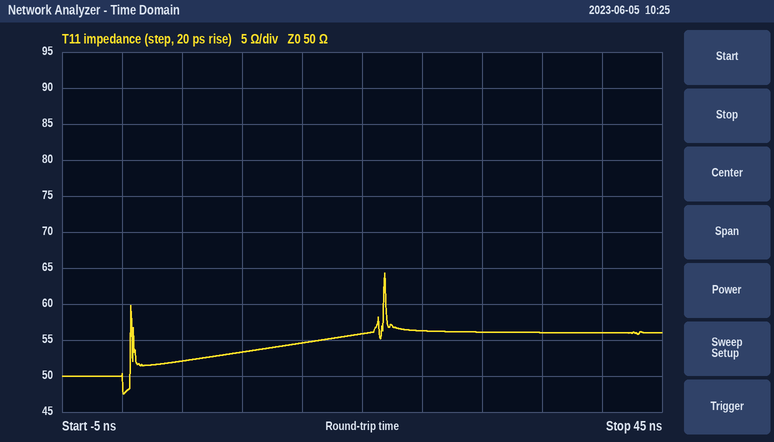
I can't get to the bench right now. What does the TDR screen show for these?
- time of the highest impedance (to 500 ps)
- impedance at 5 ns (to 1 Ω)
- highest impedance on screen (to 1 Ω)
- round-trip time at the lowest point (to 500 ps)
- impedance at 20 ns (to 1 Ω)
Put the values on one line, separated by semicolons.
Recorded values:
22.0 ns; 52 Ω; 64 Ω; 0.0 ns; 56 Ω
